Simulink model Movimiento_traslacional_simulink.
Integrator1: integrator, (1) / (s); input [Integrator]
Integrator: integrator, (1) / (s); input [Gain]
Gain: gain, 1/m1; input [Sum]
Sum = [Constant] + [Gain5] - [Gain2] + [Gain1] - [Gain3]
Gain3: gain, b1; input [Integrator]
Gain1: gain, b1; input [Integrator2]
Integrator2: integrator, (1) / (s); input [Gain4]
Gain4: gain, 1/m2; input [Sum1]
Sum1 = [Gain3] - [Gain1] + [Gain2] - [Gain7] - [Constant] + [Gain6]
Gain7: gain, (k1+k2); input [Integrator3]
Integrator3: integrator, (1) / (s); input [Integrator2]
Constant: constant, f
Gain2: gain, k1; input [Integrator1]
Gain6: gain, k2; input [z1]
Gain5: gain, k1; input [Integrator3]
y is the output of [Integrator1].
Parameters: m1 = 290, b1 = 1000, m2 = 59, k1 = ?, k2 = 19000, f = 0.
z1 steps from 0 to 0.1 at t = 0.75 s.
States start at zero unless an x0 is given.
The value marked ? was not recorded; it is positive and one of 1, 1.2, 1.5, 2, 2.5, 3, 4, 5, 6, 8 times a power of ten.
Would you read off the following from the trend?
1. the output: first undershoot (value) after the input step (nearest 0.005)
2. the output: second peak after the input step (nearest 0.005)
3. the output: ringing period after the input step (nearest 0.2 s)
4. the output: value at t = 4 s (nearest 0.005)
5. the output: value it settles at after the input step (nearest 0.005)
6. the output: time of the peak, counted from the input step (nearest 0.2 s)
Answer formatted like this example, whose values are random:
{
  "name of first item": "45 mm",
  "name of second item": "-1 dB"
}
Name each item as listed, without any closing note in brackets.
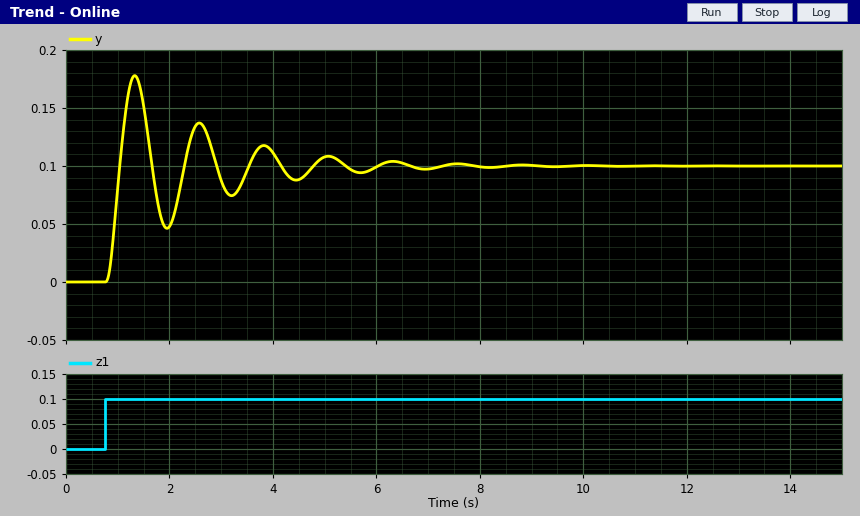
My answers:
{
  "the output: first undershoot (value) after the input step": "0.045",
  "the output: second peak after the input step": "0.135",
  "the output: ringing period after the input step": "1.2 s",
  "the output: value at t = 4 s": "0.110",
  "the output: value it settles at after the input step": "0.100",
  "the output: time of the peak, counted from the input step": "0.6 s"
}
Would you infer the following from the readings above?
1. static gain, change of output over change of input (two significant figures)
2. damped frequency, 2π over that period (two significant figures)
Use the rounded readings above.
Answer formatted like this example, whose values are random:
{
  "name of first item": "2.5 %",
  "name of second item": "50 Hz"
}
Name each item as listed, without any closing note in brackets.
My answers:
{
  "static gain, change of output over change of input": "1.0",
  "damped frequency, 2π over that period": "5.2 rad/s"
}
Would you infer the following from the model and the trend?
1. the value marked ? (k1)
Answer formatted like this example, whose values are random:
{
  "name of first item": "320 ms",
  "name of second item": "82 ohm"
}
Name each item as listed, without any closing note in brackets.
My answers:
{
  "the value marked ?": "12000"
}
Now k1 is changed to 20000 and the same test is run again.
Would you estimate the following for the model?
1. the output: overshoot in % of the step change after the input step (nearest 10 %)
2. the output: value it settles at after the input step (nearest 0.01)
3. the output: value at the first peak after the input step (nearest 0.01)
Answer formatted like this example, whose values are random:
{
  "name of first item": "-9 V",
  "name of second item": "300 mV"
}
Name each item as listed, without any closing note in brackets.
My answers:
{
  "the output: overshoot in % of the step change after the input step": "90 %",
  "the output: value it settles at after the input step": "0.10",
  "the output: value at the first peak after the input step": "0.19"
}
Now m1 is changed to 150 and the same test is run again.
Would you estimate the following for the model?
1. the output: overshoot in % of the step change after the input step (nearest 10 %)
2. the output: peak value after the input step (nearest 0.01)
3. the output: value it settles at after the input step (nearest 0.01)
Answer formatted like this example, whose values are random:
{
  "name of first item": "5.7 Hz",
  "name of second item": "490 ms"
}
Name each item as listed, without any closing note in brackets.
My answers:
{
  "the output: overshoot in % of the step change after the input step": "80 %",
  "the output: peak value after the input step": "0.18",
  "the output: value it settles at after the input step": "0.10"
}
